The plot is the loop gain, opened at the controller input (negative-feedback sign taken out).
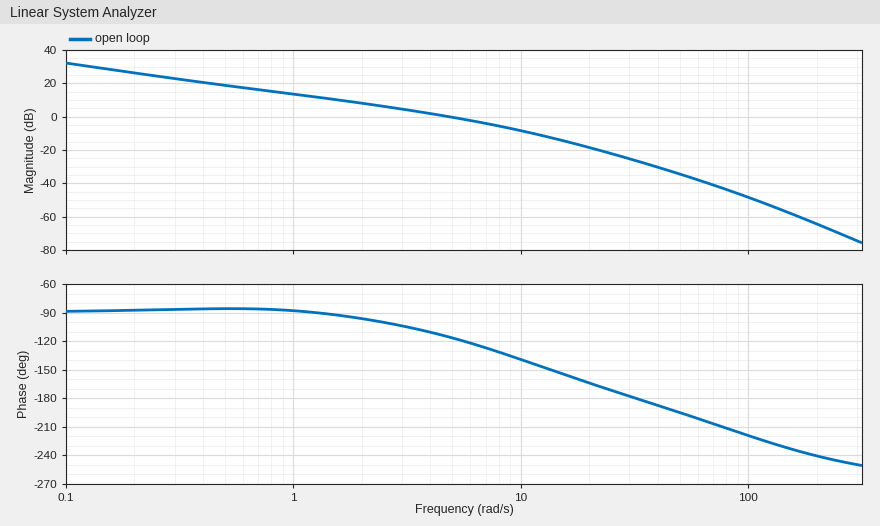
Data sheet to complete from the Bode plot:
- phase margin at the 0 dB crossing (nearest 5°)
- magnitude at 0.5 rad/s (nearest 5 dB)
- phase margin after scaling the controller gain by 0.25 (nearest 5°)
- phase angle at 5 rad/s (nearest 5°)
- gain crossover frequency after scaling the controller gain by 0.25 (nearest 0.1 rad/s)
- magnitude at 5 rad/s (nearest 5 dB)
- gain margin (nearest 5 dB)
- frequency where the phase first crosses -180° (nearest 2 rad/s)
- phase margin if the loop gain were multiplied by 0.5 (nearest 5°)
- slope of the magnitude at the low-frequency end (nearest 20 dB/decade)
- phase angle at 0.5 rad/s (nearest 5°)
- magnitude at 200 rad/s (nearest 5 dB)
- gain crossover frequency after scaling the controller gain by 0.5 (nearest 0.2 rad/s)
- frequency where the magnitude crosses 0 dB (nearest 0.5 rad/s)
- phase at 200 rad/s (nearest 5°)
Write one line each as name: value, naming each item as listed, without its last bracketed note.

phase margin at the 0 dB crossing: 65°
magnitude at 0.5 rad/s: 20 dB
phase margin after scaling the controller gain by 0.25: 90°
phase angle at 5 rad/s: -115°
gain crossover frequency after scaling the controller gain by 0.25: 1.2 rad/s
magnitude at 5 rad/s: 0 dB
gain margin: 25 dB
frequency where the phase first crosses -180°: 32 rad/s
phase margin if the loop gain were multiplied by 0.5: 80°
slope of the magnitude at the low-frequency end: -20 dB/decade
phase angle at 0.5 rad/s: -85°
magnitude at 200 rad/s: -65 dB
gain crossover frequency after scaling the controller gain by 0.5: 2.6 rad/s
frequency where the magnitude crosses 0 dB: 5.0 rad/s
phase at 200 rad/s: -240°
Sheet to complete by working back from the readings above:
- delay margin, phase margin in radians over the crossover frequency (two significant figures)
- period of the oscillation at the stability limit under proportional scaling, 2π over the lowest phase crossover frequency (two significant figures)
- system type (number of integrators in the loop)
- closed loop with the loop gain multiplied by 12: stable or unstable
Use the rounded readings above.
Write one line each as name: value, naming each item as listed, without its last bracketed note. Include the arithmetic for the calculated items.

delay margin, phase margin in radians over the crossover frequency: 65 × π / 180 / 5 = 0.23 s
period of the oscillation at the stability limit under proportional scaling, 2π over the lowest phase crossover frequency: 2π / 32 = 0.20 s
system type: 1
closed loop with the loop gain multiplied by 12: stable or unstable: stable
